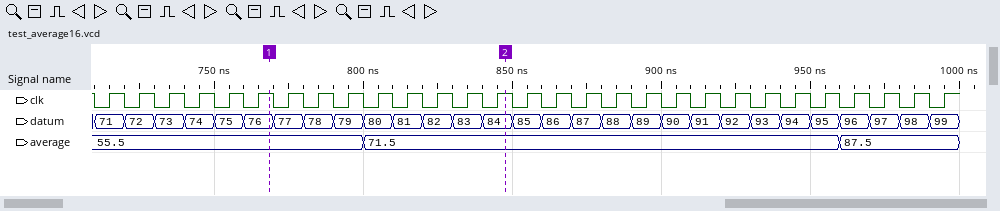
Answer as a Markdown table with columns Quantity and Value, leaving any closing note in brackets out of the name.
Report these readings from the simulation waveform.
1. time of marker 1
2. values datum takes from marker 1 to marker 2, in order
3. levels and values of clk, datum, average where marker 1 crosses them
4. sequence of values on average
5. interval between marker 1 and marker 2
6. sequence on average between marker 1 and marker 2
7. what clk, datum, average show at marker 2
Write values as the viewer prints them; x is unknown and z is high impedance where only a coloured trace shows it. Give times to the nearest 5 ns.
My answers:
| Quantity | Value |
|---|---|
| time of marker 1 | 770 ns |
| values datum takes from marker 1 to marker 2, in order | 76, 77, 78, 79, 80, 81, 82, 83, 84 |
| levels and values of clk, datum, average where marker 1 crosses them | clk=1, datum=76, average=55.5 |
| sequence of values on average | 55.5, 71.5, 87.5 |
| interval between marker 1 and marker 2 | 80 ns |
| sequence on average between marker 1 and marker 2 | 55.5, 71.5 |
| what clk, datum, average show at marker 2 | clk=1, datum=84, average=71.5 |
